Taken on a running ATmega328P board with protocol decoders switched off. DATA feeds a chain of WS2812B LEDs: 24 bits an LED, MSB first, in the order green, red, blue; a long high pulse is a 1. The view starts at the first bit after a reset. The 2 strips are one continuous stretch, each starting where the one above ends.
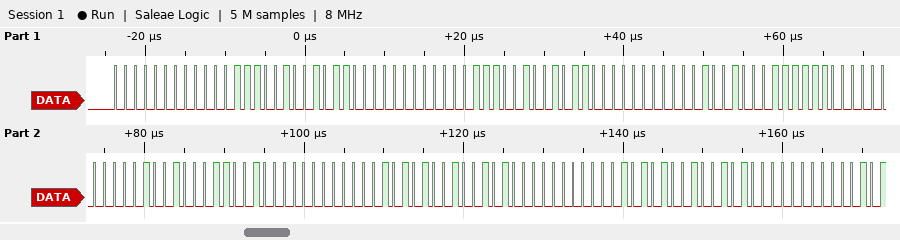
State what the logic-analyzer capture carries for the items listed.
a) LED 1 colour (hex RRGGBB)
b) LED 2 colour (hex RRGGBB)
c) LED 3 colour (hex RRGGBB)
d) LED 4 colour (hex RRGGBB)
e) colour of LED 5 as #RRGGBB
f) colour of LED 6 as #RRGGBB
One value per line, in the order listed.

#0E004B
#0E004B
#12003F
#120032
#150025
#150025
